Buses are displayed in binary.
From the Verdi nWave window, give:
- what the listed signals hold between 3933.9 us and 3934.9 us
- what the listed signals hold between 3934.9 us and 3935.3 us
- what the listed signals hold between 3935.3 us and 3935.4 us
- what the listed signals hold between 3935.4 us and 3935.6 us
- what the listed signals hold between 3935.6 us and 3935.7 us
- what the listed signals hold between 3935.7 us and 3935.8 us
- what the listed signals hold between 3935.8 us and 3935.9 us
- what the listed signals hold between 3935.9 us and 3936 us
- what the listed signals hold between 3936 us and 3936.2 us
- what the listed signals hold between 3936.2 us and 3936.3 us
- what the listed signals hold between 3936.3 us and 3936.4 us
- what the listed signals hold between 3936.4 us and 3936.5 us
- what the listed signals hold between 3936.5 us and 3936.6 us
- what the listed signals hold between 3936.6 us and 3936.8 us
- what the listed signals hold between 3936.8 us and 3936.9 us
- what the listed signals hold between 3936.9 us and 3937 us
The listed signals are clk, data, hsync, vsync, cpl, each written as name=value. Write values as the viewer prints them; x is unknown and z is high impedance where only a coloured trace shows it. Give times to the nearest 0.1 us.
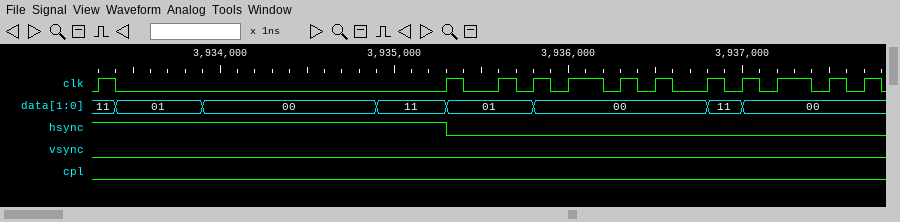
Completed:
clk=0, data=00, hsync=1, vsync=0, cpl=0
clk=0, data=11, hsync=1, vsync=0, cpl=0
clk=1, data=01, hsync=0, vsync=0, cpl=0
clk=0, data=01, hsync=0, vsync=0, cpl=0
clk=1, data=01, hsync=0, vsync=0, cpl=0
clk=0, data=01, hsync=0, vsync=0, cpl=0
clk=1, data=00, hsync=0, vsync=0, cpl=0
clk=0, data=00, hsync=0, vsync=0, cpl=0
clk=1, data=00, hsync=0, vsync=0, cpl=0
clk=0, data=00, hsync=0, vsync=0, cpl=0
clk=1, data=00, hsync=0, vsync=0, cpl=0
clk=0, data=00, hsync=0, vsync=0, cpl=0
clk=1, data=00, hsync=0, vsync=0, cpl=0
clk=0, data=00, hsync=0, vsync=0, cpl=0
clk=1, data=11, hsync=0, vsync=0, cpl=0
clk=0, data=11, hsync=0, vsync=0, cpl=0
